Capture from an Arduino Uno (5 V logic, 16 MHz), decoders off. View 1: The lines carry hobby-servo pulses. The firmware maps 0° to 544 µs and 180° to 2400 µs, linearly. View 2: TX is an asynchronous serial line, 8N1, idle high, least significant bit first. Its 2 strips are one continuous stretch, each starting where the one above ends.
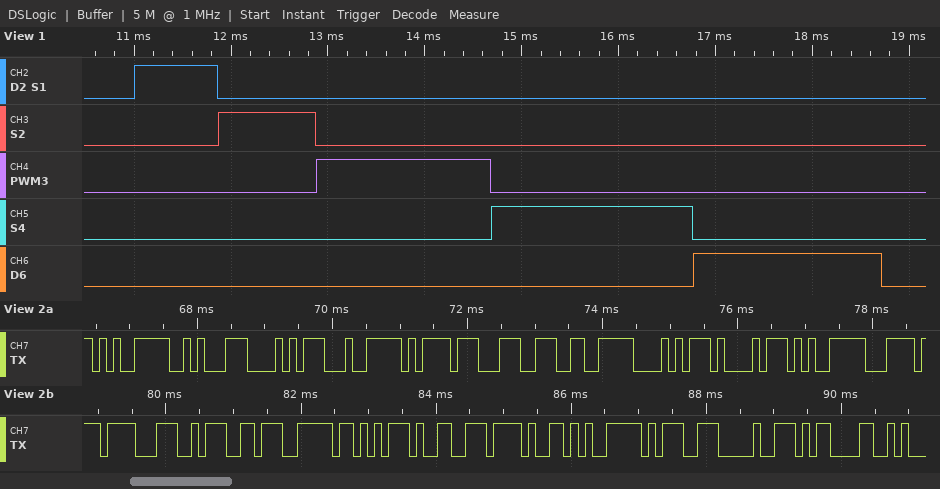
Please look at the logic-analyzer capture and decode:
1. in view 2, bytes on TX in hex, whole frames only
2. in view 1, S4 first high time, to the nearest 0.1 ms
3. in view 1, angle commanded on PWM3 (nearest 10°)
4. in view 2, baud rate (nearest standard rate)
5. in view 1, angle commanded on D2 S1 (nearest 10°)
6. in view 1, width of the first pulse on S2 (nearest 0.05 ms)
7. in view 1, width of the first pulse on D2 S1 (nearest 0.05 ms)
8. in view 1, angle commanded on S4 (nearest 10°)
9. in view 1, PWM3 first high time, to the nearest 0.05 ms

0xE5 0x8A 0xA8 0xE4 0xBD 0x9C 0xE6 0xA8 0xA1 0xE5 0xBC 0x8F 0x3A 0xE7 0xAB 0x99 0x2F 0xE5 0x9D 0x90 0x0D
2.1 ms
120°
9600 baud
30°
1.00 ms
0.85 ms
150°
1.80 ms
